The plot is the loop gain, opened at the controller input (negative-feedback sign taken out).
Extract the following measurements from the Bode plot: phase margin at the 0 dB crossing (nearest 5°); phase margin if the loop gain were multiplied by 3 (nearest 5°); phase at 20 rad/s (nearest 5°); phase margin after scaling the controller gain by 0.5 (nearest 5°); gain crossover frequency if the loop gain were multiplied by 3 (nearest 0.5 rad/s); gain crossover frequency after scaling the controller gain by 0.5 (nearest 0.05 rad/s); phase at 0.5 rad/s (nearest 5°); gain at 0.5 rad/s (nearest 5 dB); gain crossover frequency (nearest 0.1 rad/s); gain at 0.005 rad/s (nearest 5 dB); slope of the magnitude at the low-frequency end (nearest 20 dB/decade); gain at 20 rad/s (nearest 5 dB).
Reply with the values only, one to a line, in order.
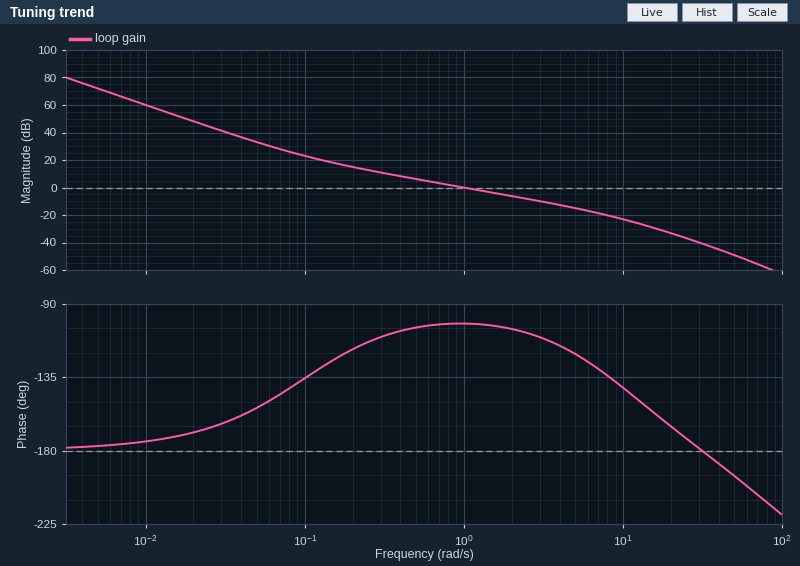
80°
70°
-165°
75°
3.0 rad/s
0.50 rad/s
-105°
5 dB
1.0 rad/s
70 dB
-40 dB/decade
-35 dB
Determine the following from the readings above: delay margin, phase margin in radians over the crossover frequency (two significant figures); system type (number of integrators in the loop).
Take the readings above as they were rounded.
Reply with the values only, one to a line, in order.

1.4 s
2
